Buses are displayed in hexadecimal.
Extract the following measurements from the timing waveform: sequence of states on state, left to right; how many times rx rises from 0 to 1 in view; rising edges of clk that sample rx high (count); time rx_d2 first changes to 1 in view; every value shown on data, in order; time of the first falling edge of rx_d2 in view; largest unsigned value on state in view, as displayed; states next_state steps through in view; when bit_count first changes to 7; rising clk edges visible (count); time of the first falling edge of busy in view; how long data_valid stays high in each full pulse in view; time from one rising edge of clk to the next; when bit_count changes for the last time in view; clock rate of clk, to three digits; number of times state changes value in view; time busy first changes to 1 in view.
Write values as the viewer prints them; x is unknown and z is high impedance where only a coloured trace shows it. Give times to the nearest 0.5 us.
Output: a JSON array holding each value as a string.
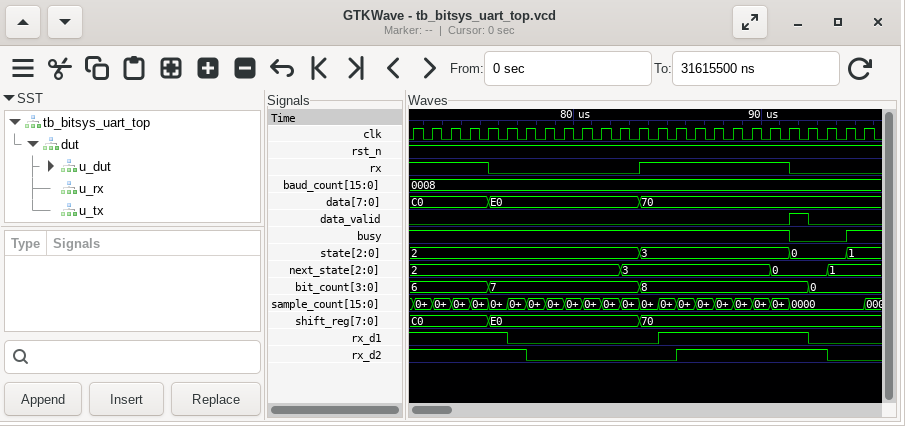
["2, 3, 0, 1", "1", "13", "85.5 us", "C0, E0, 70", "77.5 us", "3", "2, 3, 0, 1", "75.5 us", "25", "91.5 us", "1 us", "1 us", "92.5 us", "1.00 MHz", "3", "94.5 us"]
